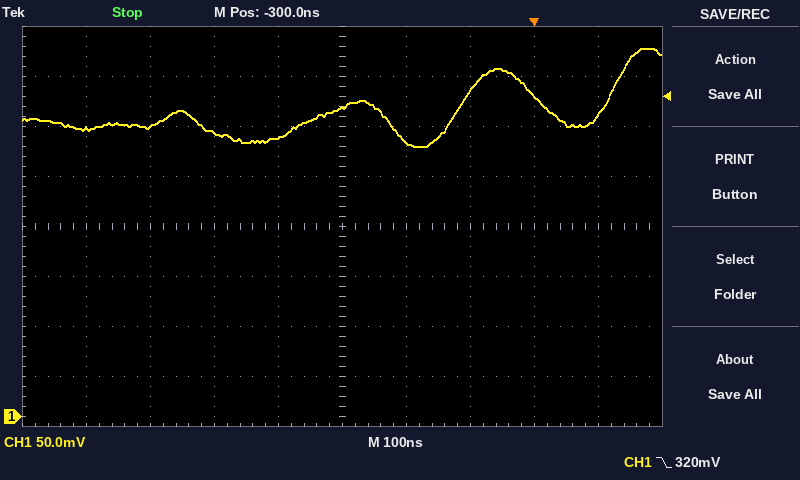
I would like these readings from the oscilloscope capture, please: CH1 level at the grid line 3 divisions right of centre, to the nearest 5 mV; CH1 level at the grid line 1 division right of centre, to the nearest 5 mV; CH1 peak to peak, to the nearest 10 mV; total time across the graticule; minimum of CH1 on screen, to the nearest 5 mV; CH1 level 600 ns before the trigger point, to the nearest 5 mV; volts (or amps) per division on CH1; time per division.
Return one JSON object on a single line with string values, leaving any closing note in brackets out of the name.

{"CH1 level at the grid line 3 divisions right of centre, to the nearest 5 mV": "320 mV", "CH1 level at the grid line 1 division right of centre, to the nearest 5 mV": "275 mV", "CH1 peak to peak, to the nearest 10 mV": "100 mV", "total time across the graticule": "1 µs", "minimum of CH1 on screen, to the nearest 5 mV": "270 mV", "CH1 level 600 ns before the trigger point, to the nearest 5 mV": "290 mV", "volts (or amps) per division on CH1": "50 mV", "time per division": "100 ns"}
